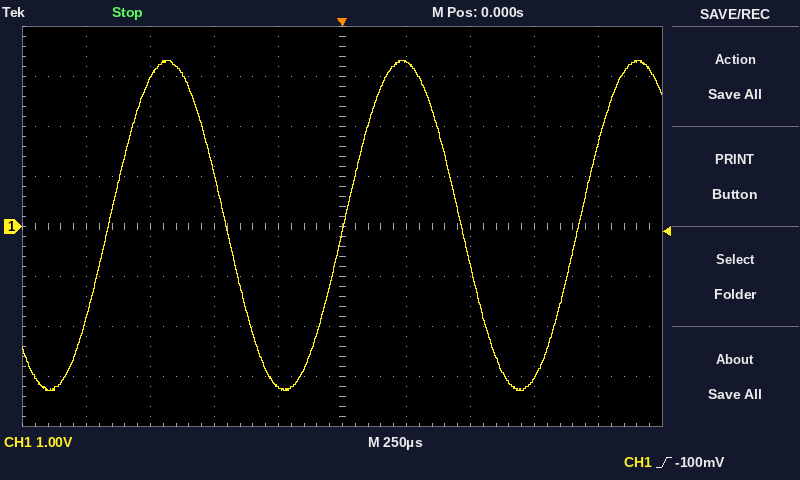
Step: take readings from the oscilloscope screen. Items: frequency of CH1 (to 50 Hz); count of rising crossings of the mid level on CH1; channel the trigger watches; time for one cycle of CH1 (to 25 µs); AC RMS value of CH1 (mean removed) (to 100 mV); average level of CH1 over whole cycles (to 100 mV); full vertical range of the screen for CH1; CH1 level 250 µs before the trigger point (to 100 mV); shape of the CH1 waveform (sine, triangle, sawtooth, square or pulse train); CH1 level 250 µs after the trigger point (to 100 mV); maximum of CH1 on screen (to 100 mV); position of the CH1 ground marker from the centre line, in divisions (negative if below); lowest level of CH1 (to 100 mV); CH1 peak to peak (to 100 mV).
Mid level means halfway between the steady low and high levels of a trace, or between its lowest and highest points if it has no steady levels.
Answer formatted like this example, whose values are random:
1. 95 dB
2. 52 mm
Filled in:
1. 1.10 kHz
2. 3
3. CH1
4. 925 µs
5. 2.3 V
6. 0.0 V
7. 8 V
8. -3.2 V
9. sine
10. 3.3 V
11. 3.3 V
12. 0.0 div
13. -3.3 V
14. 6.6 V
